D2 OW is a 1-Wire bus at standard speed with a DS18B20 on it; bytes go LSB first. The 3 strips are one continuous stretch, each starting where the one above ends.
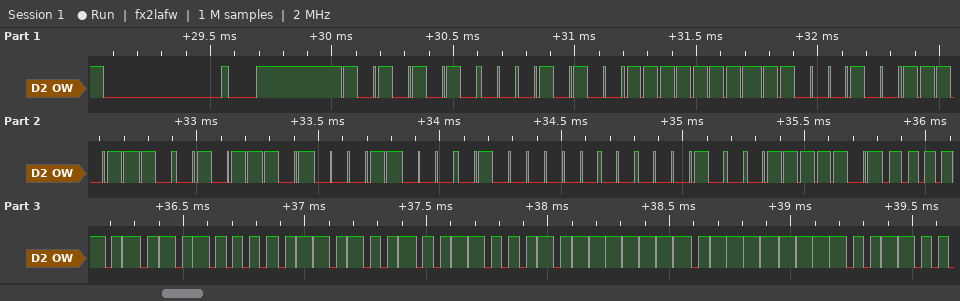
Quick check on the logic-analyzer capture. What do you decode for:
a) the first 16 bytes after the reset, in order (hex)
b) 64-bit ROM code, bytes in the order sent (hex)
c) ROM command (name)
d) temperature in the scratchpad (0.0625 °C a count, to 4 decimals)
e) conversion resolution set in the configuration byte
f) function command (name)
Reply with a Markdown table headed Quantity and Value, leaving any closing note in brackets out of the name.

| Quantity | Value |
|---|---|
| the first 16 bytes after the reset, in order | 55 28 FF 23 77 BA 18 02 20 BE 50 05 4B 46 7F FF |
| 64-bit ROM code, bytes in the order sent | 28 FF 23 77 BA 18 02 20 |
| ROM command | Match ROM |
| temperature in the scratchpad | 85.0000 °C |
| conversion resolution set in the configuration byte | 12 bits |
| function command | Read Scratchpad |
